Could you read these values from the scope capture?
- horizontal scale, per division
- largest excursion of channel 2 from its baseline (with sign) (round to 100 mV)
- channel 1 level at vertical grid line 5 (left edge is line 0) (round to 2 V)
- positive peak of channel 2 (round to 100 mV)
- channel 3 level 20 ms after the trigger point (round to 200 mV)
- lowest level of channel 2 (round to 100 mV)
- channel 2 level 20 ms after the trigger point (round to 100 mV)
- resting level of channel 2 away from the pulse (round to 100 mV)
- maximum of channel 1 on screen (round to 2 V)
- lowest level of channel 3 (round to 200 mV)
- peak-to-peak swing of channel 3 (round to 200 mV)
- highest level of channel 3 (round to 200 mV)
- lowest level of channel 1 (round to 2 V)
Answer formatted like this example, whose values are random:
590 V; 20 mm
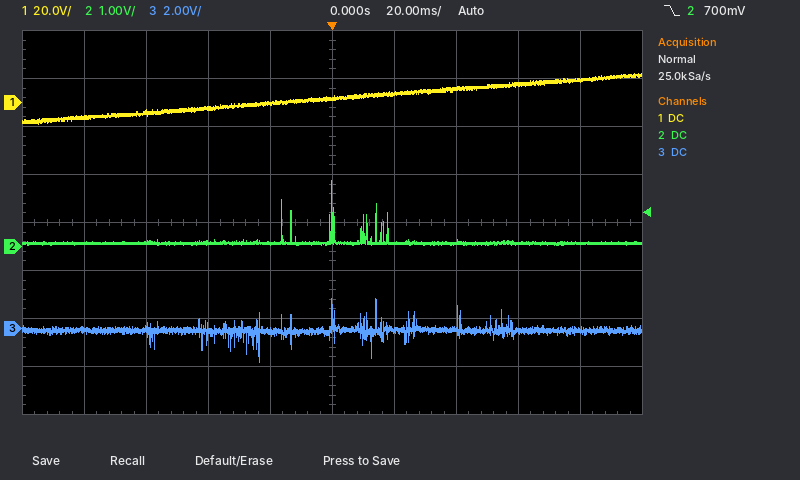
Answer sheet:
20 ms; +1.3 V; 2 V; 1.4 V; 0.0 V; 0.0 V; 100 mV; 100 mV; 12 V; -1.4 V; 2.6 V; 1.2 V; -8 V
